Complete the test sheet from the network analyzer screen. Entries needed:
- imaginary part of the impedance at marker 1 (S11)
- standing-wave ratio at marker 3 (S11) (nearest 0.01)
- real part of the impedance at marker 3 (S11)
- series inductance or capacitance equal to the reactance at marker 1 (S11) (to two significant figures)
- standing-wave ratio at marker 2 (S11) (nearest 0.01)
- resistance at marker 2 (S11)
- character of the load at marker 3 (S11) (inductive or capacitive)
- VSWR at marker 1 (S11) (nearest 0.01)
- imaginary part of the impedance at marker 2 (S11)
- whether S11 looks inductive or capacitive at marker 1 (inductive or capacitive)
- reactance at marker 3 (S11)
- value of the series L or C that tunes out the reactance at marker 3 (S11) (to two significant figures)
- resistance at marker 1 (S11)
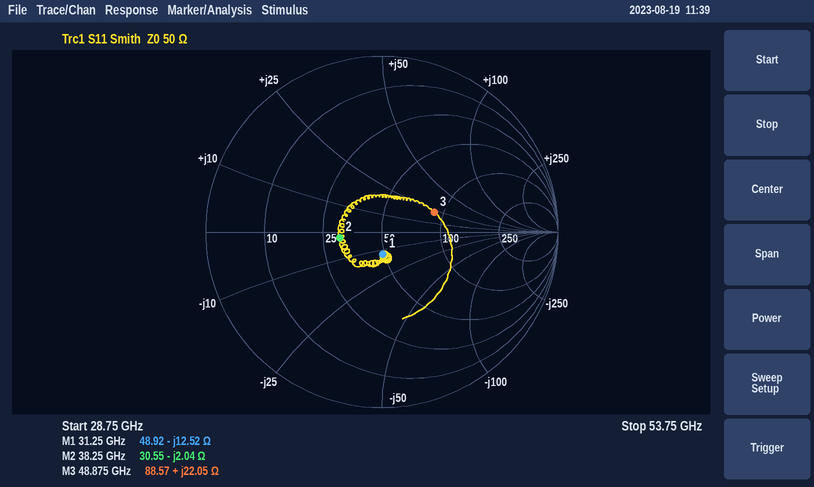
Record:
-12.52 Ω
1.93
88.57 Ω
410 fF
1.64
30.55 Ω
inductive
1.29
-2.04 Ω
capacitive
+22.05 Ω
150 fF
48.92 Ω
